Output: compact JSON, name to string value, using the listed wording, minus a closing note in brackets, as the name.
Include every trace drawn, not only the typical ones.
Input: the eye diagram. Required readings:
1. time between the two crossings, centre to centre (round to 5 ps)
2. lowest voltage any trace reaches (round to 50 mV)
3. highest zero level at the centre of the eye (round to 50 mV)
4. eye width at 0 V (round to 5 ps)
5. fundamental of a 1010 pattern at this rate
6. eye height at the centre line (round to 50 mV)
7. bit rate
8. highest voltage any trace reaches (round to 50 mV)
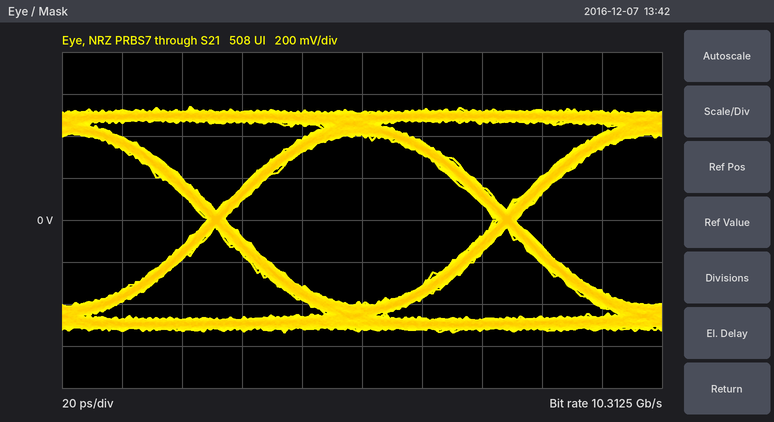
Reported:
{"time between the two crossings, centre to centre": "95 ps", "lowest voltage any trace reaches": "-550 mV", "highest zero level at the centre of the eye": "-400 mV", "eye width at 0 V": "90 ps", "fundamental of a 1010 pattern at this rate": "5.15625 GHz", "eye height at the centre line": "800 mV", "bit rate": "10.3125 Gb/s", "highest voltage any trace reaches": "550 mV"}
